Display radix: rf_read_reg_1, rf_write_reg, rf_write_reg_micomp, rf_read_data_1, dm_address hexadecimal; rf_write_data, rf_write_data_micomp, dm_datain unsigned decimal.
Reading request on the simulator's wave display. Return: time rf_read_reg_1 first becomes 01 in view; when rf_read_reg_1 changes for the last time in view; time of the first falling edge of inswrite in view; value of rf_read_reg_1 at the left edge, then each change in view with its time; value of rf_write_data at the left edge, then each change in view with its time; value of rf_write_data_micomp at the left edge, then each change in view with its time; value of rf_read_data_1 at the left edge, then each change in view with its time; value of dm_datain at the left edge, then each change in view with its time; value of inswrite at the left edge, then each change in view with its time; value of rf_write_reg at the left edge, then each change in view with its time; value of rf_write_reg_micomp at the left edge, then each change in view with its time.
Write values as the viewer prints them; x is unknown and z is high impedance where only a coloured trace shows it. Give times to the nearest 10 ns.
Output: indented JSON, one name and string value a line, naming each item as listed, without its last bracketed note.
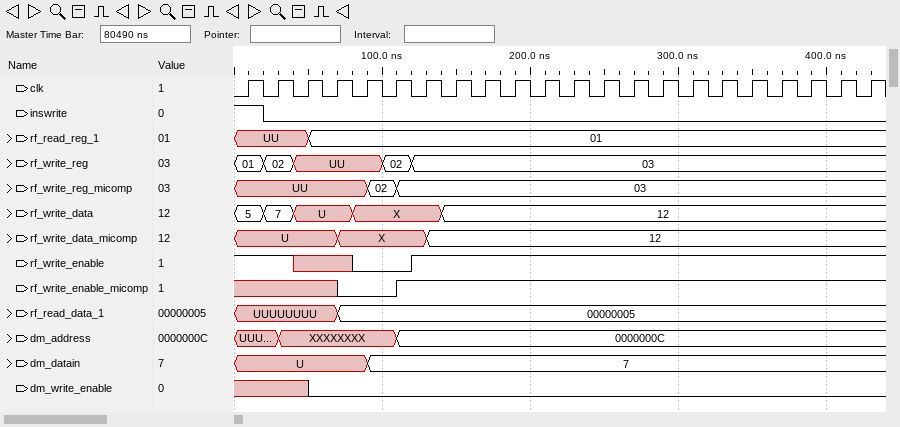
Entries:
{
  "time rf_read_reg_1 first becomes 01 in view": "50 ns",
  "when rf_read_reg_1 changes for the last time in view": "50 ns",
  "time of the first falling edge of inswrite in view": "20 ns",
  "value of rf_read_reg_1 at the left edge, then each change in view with its time": "UU, 01 at 50 ns",
  "value of rf_write_data at the left edge, then each change in view with its time": "5, 7 at 20 ns, U at 40 ns, X at 80 ns, 12 at 140 ns",
  "value of rf_write_data_micomp at the left edge, then each change in view with its time": "U, X at 70 ns, 12 at 130 ns",
  "value of rf_read_data_1 at the left edge, then each change in view with its time": "UUUUUUUU, 00000005 at 70 ns",
  "value of dm_datain at the left edge, then each change in view with its time": "U, 7 at 90 ns",
  "value of inswrite at the left edge, then each change in view with its time": "1, 0 at 20 ns",
  "value of rf_write_reg at the left edge, then each change in view with its time": "01, 02 at 20 ns, UU at 40 ns, 02 at 100 ns, 03 at 120 ns",
  "value of rf_write_reg_micomp at the left edge, then each change in view with its time": "UU, 02 at 90 ns, 03 at 110 ns"
}
